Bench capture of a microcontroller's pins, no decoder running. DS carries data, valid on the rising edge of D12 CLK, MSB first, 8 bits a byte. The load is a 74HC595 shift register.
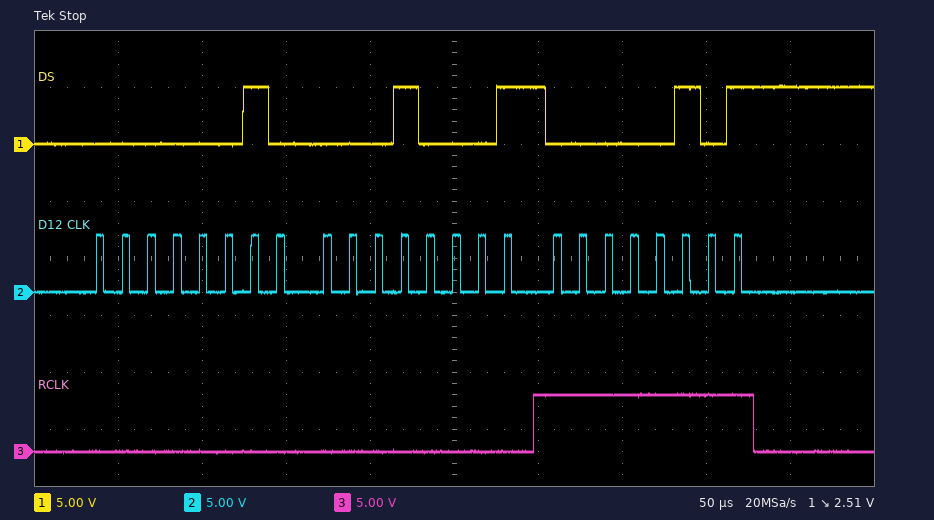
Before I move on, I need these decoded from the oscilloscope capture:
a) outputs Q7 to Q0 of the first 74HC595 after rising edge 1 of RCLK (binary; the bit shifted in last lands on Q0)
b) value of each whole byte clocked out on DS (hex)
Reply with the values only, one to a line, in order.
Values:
00010001
02 11 05
